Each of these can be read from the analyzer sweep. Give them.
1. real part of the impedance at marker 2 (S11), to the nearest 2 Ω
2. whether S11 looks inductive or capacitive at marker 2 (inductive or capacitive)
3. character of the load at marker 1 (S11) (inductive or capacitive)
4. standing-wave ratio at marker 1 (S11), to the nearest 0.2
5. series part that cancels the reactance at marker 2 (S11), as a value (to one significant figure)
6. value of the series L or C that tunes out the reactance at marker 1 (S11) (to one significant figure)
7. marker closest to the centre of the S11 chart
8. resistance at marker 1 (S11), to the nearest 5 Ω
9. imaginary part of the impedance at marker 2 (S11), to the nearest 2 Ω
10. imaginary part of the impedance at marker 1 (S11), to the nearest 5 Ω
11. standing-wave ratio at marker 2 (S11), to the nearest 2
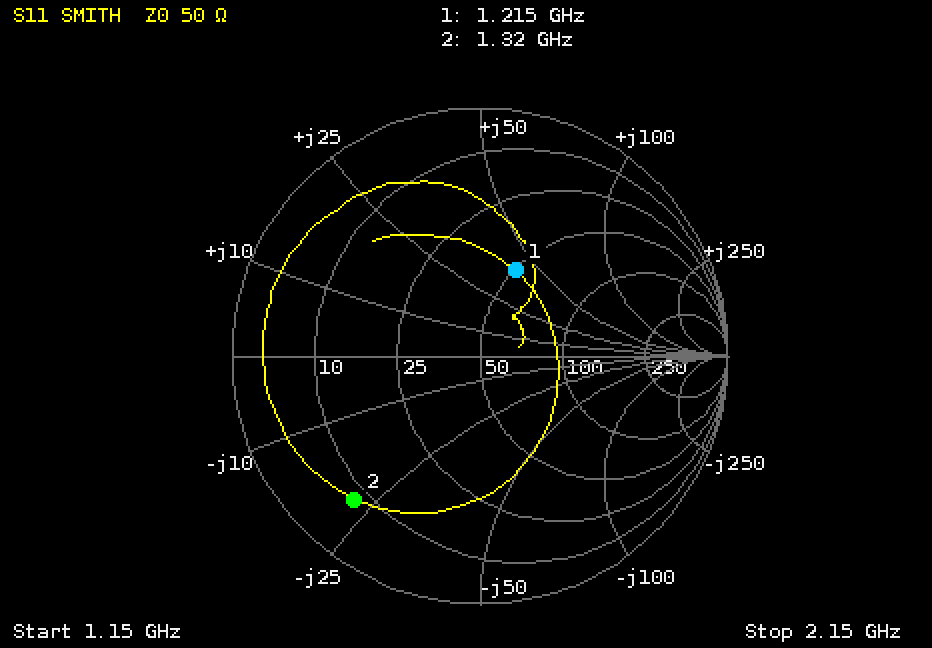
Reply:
8 Ω
capacitive
inductive
2.2
3 nH
3 pF
marker 1
50 Ω
-22 Ω
+40 Ω
8
